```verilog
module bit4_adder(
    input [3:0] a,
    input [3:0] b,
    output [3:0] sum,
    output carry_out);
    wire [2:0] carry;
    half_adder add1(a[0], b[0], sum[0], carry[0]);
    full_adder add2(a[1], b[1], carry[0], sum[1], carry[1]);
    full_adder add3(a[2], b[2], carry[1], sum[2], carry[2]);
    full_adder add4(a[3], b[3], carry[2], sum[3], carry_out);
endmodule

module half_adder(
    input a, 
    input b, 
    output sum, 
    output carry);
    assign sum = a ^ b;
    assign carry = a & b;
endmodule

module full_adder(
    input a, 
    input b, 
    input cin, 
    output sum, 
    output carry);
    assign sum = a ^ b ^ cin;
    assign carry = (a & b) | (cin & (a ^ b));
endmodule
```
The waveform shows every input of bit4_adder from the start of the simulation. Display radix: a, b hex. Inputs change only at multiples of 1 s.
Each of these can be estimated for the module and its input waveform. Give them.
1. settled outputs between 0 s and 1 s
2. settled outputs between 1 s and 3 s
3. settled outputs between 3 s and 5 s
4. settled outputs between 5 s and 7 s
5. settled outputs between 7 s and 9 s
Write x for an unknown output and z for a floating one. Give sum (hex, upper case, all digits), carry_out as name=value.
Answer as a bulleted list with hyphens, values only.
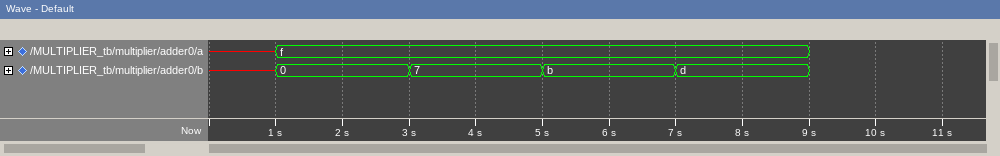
- sum=x, carry_out=x
- sum=F, carry_out=0
- sum=6, carry_out=1
- sum=A, carry_out=1
- sum=C, carry_out=1
